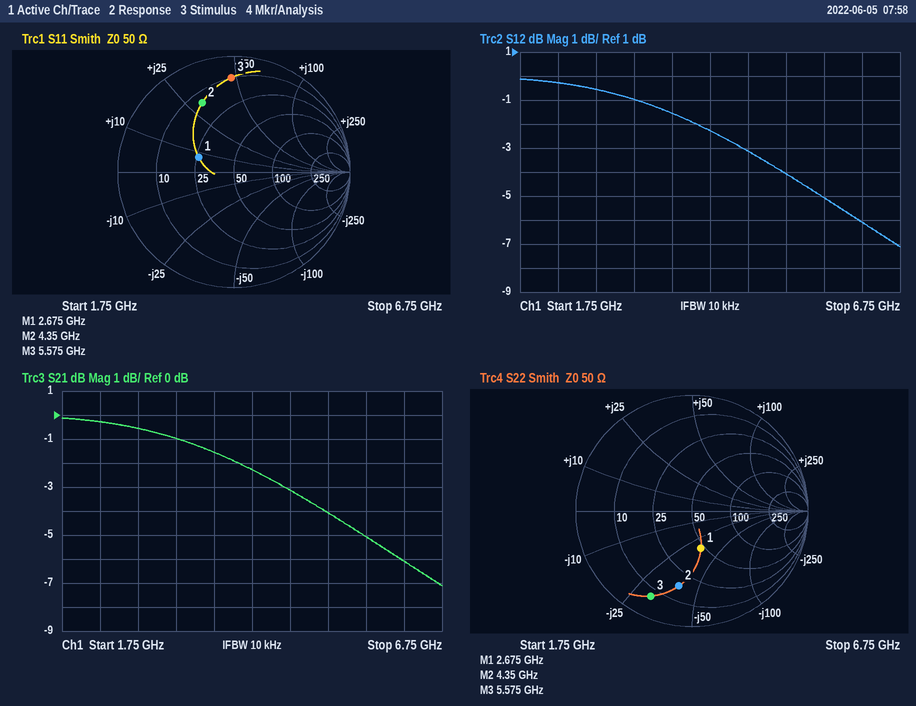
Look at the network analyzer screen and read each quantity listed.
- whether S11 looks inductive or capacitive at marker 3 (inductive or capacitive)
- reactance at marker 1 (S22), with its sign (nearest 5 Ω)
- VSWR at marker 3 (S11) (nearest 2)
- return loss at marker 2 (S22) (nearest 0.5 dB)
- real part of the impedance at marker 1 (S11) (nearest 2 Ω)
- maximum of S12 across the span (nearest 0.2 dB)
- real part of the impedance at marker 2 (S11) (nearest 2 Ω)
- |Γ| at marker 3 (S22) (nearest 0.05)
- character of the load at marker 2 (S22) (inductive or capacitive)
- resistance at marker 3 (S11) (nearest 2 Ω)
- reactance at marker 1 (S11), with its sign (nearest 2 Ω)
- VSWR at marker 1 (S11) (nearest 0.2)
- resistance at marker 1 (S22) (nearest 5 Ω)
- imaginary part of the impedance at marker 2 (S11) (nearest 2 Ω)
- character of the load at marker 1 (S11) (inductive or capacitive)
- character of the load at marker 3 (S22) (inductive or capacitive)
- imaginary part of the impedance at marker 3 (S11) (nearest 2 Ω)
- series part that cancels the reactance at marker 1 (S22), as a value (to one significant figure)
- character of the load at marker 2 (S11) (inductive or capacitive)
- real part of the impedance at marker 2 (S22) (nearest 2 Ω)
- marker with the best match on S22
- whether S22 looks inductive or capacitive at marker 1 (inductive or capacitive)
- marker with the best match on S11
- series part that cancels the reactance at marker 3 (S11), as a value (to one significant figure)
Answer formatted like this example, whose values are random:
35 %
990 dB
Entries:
inductive
-35 Ω
10
3.5 dB
26 Ω
-0.2 dB
14 Ω
0.80
capacitive
10 Ω
+8 Ω
2.0
45 Ω
+30 Ω
inductive
capacitive
+48 Ω
2 nH
inductive
18 Ω
marker 1
capacitive
marker 1
600 fF
